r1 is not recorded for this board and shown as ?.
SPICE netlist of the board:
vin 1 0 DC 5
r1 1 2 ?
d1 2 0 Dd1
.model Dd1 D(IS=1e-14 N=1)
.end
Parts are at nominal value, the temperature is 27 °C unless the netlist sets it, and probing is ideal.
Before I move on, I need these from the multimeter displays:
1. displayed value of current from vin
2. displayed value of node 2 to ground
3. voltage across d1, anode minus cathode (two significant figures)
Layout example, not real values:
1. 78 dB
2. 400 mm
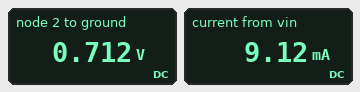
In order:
1. 9.12 mA
2. 0.712 V
3. 710 mV
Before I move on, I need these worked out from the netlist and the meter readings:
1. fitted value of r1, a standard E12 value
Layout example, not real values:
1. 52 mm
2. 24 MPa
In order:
1. 470 Ω
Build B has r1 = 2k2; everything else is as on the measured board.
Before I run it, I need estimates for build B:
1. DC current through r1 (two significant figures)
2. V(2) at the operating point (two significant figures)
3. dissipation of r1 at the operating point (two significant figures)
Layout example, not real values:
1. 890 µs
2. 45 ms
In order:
1. 2.0 mA
2. 670 mV
3. 8.5 mW
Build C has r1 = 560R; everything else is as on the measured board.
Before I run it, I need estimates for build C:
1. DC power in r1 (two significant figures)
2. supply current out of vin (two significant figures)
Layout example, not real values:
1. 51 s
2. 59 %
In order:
1. 33 mW
2. 7.7 mA
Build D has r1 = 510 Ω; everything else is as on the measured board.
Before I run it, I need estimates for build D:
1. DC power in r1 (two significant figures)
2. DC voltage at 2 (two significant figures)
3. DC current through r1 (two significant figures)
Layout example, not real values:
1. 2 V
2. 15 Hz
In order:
1. 36 mW
2. 710 mV
3. 8.4 mA
